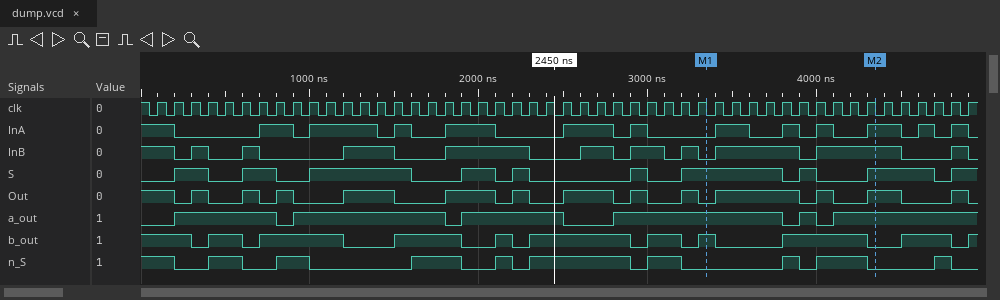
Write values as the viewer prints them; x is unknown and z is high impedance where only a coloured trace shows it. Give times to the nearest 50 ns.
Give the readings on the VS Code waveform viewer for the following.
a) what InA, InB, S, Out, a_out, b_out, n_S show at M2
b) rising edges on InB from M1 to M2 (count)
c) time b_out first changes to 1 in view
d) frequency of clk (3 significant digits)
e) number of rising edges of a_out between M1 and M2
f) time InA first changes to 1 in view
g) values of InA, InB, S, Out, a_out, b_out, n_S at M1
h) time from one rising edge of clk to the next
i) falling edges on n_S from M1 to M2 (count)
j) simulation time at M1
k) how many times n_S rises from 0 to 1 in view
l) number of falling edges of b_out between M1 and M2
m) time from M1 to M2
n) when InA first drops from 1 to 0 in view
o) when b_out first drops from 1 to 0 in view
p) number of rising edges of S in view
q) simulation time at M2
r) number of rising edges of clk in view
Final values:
InA=1, InB=1, S=1, Out=1, a_out=1, b_out=0, n_S=0
2
400 ns
10.0 MHz
2
700 ns
InA=0, InB=0, S=1, Out=0, a_out=1, b_out=1, n_S=0
100 ns
2
3350 ns
9
2
1000 ns
200 ns
300 ns
10
4350 ns
49
